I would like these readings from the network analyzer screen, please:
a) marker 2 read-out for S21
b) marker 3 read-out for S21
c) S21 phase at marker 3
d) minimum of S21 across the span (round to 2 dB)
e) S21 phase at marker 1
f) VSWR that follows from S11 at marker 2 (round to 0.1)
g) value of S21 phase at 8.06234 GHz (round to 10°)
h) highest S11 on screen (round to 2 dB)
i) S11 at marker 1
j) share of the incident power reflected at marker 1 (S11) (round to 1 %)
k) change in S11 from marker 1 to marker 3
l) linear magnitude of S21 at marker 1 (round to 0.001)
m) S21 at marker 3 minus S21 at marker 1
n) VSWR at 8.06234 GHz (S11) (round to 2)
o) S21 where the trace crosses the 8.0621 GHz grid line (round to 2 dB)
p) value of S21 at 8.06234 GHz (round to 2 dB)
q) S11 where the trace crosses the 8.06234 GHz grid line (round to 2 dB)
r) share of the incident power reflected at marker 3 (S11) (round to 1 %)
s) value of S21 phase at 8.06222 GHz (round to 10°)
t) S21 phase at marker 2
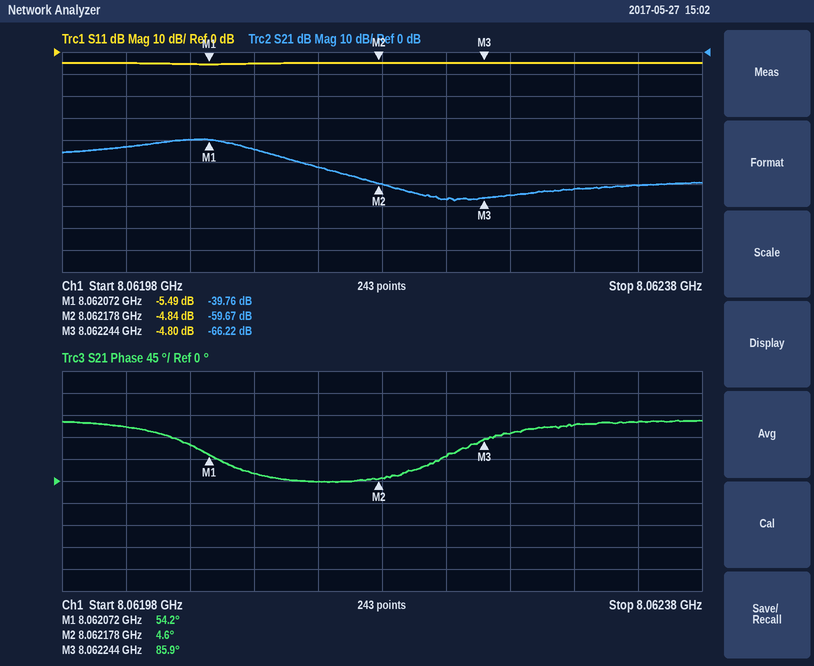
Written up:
-59.67 dB
-66.22 dB
85.9°
-68 dB
54.2°
3.7
120°
-4 dB
-5.49 dB
28 %
0.69 dB
0.010
-26.46 dB
4
-44 dB
-60 dB
-4 dB
33 %
50°
4.6°
